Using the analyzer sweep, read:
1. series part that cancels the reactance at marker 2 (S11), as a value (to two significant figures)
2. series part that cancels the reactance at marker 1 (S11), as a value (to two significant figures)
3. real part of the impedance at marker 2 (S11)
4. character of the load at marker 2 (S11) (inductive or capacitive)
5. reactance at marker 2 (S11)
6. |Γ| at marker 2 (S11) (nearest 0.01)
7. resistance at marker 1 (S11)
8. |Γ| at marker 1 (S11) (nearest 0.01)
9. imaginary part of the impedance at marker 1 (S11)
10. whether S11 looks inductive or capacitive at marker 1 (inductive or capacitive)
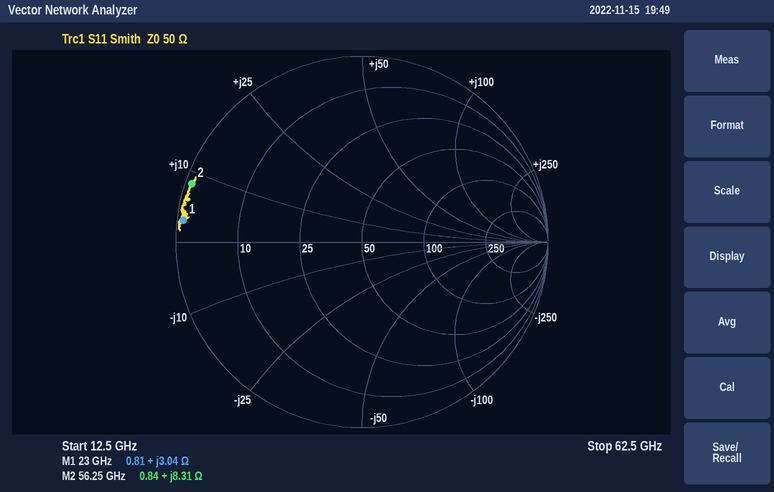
340 fF
2.3 pF
0.84 Ω
inductive
+8.31 Ω
0.97
0.81 Ω
0.97
+3.04 Ω
inductive
